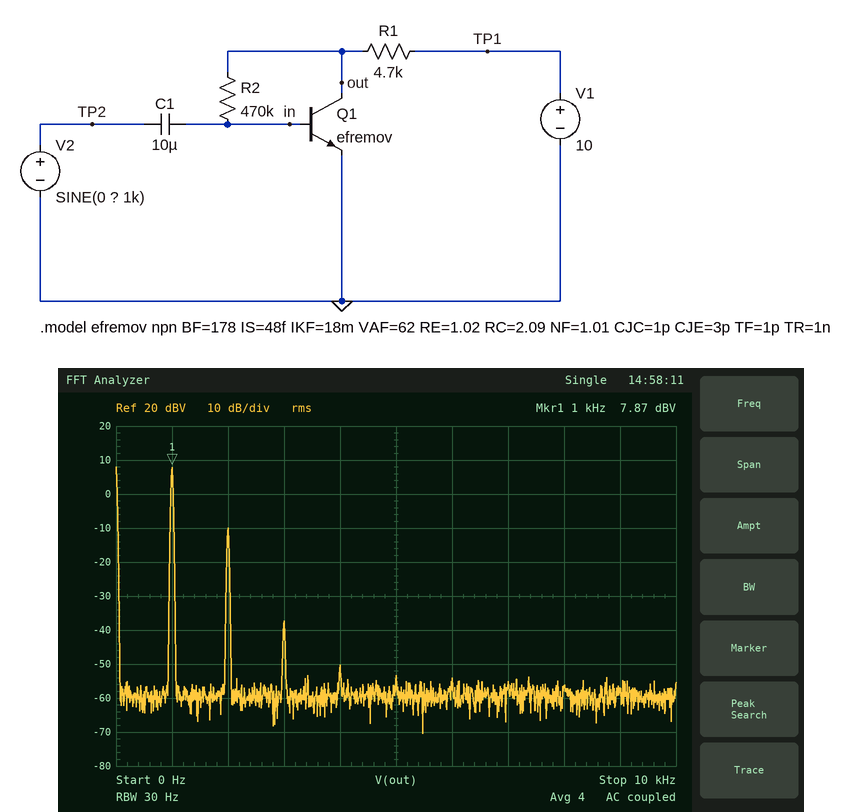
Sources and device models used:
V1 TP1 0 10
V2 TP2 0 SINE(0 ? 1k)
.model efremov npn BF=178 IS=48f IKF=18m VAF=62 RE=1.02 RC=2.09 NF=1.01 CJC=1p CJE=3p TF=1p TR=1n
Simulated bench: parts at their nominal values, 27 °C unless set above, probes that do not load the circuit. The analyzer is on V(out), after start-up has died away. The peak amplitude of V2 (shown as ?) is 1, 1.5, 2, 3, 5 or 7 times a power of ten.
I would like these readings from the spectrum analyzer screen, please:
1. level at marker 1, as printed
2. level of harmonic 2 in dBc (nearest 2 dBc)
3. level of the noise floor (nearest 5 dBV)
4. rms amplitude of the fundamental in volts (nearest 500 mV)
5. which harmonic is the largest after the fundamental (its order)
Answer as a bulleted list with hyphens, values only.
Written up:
- 7.87 dBV
- -18 dBc
- -60 dBV
- 2.5 V
- 2
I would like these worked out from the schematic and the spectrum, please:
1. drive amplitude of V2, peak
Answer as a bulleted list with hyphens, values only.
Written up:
- 20 mV
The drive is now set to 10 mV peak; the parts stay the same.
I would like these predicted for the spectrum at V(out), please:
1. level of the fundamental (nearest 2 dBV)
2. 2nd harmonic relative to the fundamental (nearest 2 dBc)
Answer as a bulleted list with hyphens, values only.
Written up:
- 2 dBV
- -24 dBc
